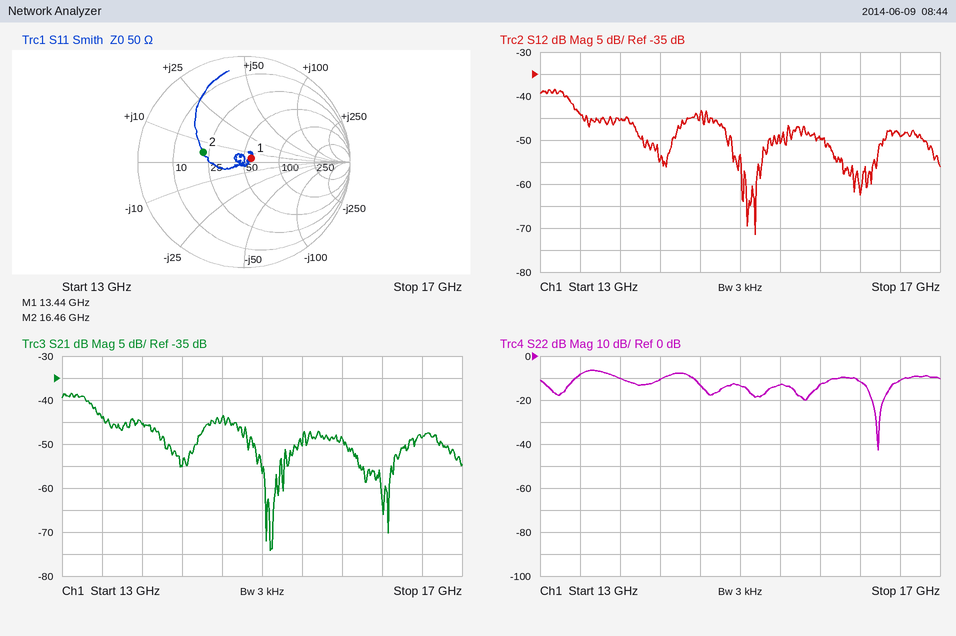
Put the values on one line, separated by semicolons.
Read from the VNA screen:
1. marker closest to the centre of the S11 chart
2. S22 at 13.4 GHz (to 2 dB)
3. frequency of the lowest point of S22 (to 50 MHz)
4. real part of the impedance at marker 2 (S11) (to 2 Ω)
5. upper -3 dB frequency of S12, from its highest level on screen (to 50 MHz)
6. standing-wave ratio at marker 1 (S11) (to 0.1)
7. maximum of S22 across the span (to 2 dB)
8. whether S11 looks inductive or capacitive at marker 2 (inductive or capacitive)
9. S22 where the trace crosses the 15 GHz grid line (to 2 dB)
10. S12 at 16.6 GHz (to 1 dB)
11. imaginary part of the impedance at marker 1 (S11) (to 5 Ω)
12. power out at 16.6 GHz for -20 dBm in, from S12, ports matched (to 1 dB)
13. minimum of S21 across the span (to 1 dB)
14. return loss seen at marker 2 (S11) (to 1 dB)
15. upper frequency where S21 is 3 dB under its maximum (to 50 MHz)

marker 1; -8 dB; 16.40 GHz; 22 Ω; 13.30 GHz; 1.2; -6 dB; inductive; -14 dB; -49 dB; +5 Ω; -69 dBm; -74 dB; 8 dB; 13.30 GHz
